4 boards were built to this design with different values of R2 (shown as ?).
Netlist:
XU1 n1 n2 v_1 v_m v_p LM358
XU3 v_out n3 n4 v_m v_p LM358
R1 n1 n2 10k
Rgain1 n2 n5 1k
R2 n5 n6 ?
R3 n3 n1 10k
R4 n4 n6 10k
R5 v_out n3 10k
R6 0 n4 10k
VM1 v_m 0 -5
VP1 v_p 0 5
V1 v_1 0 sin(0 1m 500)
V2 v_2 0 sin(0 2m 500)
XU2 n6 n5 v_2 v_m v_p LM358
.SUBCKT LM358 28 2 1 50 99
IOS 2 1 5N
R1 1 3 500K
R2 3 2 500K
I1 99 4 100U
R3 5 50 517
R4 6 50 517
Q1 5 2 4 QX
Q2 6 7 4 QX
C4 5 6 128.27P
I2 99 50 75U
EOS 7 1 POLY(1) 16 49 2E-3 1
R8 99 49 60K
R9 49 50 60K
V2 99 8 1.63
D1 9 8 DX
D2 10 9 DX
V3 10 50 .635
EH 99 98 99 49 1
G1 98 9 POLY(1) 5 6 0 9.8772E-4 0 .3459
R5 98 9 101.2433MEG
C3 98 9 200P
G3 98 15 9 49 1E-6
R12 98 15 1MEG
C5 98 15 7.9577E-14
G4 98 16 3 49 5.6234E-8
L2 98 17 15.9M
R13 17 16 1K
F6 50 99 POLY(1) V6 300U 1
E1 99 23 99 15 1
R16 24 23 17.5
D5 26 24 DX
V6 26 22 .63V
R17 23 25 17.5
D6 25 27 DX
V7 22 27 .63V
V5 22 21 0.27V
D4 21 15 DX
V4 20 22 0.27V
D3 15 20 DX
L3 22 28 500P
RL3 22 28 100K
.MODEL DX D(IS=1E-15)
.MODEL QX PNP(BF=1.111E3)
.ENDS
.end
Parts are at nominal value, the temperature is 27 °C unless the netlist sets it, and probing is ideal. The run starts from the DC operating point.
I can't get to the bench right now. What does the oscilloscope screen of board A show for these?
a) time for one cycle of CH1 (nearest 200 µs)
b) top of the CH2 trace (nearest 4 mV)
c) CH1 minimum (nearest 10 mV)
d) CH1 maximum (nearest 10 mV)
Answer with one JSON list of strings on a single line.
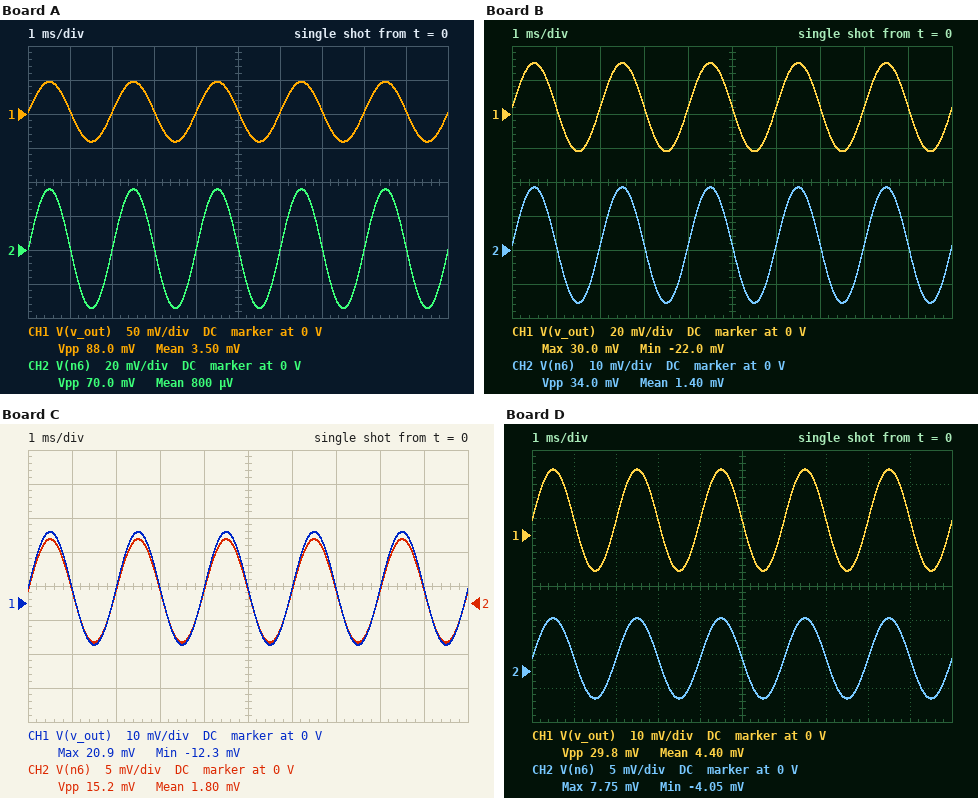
["2.0 ms", "36 mV", "-40 mV", "50 mV"]
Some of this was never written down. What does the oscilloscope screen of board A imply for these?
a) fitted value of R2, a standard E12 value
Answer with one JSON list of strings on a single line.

["33 kΩ"]
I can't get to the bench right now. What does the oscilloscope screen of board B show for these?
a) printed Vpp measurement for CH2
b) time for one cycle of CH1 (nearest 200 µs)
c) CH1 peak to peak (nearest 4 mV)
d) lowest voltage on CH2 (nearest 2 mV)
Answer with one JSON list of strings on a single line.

["34.0 mV", "2.0 ms", "52 mV", "-16 mV"]
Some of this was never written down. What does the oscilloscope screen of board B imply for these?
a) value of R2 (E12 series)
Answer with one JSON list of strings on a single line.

["15 kΩ"]
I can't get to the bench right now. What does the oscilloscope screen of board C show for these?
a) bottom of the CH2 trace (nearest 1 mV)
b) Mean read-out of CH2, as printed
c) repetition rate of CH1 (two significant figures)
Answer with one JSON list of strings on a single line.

["-6 mV", "1.80 mV", "500 Hz"]
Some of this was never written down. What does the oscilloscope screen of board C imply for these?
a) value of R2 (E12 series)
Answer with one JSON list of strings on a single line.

["5.6 kΩ"]
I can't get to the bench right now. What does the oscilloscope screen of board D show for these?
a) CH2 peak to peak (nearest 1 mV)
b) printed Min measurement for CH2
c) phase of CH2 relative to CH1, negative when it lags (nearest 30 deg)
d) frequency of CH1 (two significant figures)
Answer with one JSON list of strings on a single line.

["12 mV", "-4.05 mV", "0 deg", "500 Hz"]
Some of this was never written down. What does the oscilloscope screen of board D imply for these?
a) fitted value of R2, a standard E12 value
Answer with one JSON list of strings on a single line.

["3.9 kΩ"]
